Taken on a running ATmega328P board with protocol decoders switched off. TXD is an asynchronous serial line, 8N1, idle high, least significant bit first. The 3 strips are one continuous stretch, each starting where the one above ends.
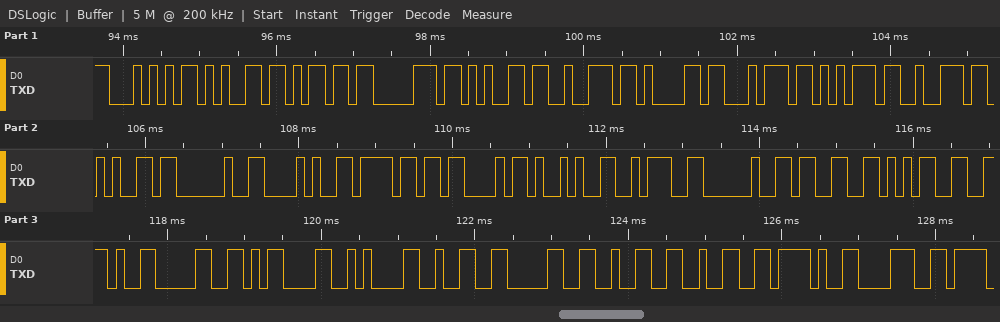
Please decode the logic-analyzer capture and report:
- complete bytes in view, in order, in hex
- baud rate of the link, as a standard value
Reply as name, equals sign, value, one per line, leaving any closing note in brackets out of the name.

complete bytes in view, in order, in hex = 54 65 6D 70 65 72 61 74 75 72 65 20 28 6F 43 29 3A 20 33 35 2E 30 0D 0A 32 30 32 32 2F 38
baud rate of the link, as a standard value = 9600 baud
